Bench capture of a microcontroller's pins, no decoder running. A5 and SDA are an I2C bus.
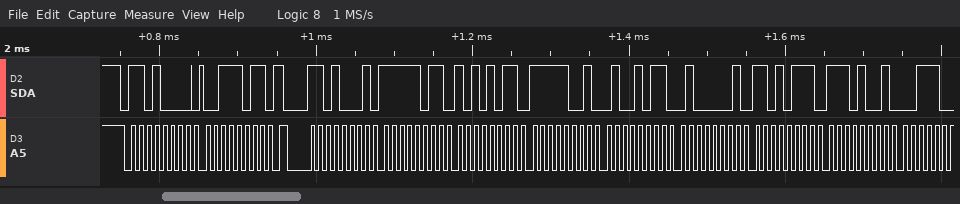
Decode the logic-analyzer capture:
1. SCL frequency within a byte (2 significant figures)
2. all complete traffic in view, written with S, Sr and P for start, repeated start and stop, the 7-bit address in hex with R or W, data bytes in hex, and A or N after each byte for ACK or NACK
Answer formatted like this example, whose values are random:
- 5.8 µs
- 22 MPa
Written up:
- 100 kHz
- S 68W A 3B A Sr 68R A FB A AB A F9 A 4B A 41 A D7 A E9 A
